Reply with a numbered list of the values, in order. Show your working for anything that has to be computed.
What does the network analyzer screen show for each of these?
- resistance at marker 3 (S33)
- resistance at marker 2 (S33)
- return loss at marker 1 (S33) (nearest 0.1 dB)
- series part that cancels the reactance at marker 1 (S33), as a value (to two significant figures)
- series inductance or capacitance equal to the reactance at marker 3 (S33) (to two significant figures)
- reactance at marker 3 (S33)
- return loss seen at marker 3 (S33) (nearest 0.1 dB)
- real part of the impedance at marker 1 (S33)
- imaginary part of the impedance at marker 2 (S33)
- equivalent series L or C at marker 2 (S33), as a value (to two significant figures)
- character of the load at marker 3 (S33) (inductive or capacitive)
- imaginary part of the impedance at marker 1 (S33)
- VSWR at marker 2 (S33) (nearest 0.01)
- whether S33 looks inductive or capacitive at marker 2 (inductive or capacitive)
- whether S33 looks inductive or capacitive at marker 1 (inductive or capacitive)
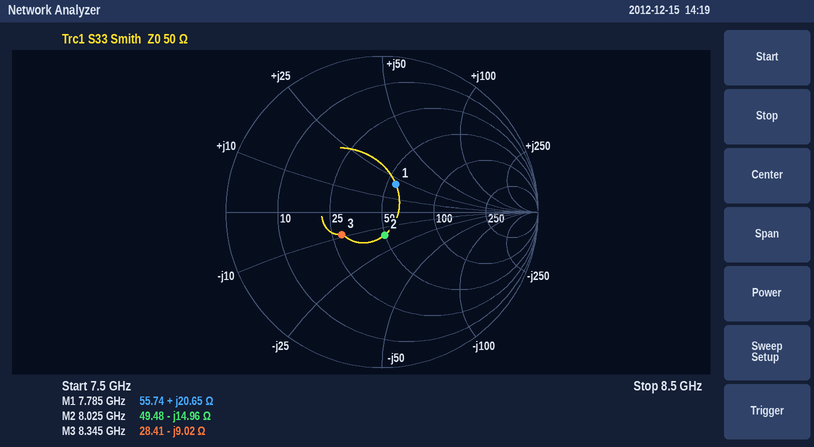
1. 28.41 Ω
2. 49.48 Ω
3. 14.0 dB
4. C = 1/(2π × 7.785 GHz × 20.65 Ω) ≈ 990 fF
5. C = 1/(2π × 8.345 GHz × 9.02 Ω) ≈ 2.1 pF
6. -9.02 Ω
7. 10.6 dB
8. 55.74 Ω
9. -14.96 Ω
10. C = 1/(2π × 8.025 GHz × 14.96 Ω) ≈ 1.3 pF
11. capacitive
12. +20.65 Ω
13. 1.35
14. capacitive
15. inductive
